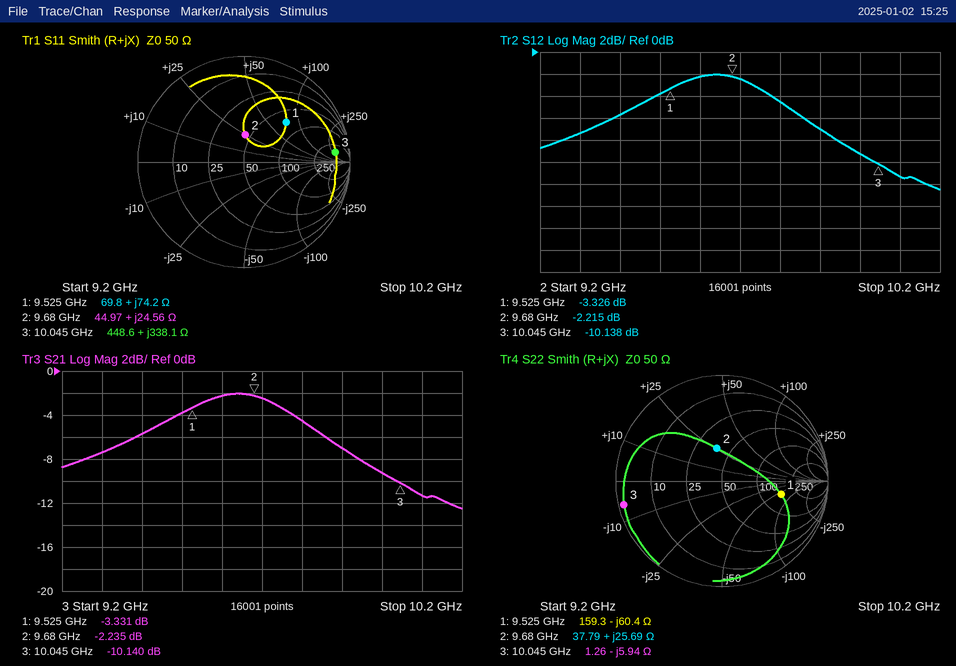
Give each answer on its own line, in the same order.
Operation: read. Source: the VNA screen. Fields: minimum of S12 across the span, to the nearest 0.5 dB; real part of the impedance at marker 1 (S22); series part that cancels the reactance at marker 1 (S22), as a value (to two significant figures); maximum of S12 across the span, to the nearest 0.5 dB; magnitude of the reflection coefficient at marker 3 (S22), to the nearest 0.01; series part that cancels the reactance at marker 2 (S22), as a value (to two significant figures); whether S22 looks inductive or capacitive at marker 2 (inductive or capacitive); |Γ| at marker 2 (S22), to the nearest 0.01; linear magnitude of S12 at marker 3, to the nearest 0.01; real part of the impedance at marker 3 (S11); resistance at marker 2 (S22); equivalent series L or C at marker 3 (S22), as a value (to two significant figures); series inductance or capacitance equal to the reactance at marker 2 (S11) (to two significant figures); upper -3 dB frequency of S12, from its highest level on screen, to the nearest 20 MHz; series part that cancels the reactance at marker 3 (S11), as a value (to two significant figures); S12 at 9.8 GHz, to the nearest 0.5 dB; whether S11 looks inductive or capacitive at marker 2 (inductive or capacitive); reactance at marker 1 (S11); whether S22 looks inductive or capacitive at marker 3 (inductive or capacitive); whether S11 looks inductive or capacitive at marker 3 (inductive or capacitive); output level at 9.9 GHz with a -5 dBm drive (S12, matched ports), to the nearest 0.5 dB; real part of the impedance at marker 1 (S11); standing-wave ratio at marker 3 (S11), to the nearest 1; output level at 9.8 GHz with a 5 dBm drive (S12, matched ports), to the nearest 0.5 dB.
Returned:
-12.5 dB
159.3 Ω
1.0 nH
-2.0 dB
0.95
640 fF
inductive
0.31
0.31
448.6 Ω
37.79 Ω
2.7 pF
400 pH
9.82 GHz
47 fF
-4.5 dB
inductive
+74.2 Ω
capacitive
inductive
-12.0 dBm
69.8 Ω
14
0.5 dBm
